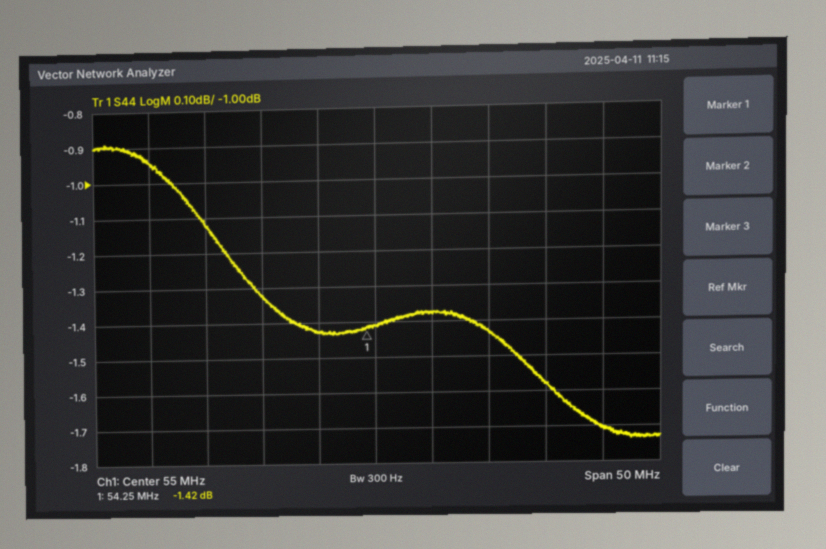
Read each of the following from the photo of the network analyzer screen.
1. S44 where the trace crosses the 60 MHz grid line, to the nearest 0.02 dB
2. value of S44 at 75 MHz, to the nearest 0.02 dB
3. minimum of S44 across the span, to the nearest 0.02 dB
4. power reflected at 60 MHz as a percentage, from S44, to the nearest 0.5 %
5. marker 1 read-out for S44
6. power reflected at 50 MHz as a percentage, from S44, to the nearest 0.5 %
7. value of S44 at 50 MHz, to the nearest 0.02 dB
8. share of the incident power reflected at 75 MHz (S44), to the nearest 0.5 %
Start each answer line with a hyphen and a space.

- -1.38 dB
- -1.70 dB
- -1.74 dB
- 73.0 %
- -1.42 dB
- 72.0 %
- -1.42 dB
- 67.5 %
